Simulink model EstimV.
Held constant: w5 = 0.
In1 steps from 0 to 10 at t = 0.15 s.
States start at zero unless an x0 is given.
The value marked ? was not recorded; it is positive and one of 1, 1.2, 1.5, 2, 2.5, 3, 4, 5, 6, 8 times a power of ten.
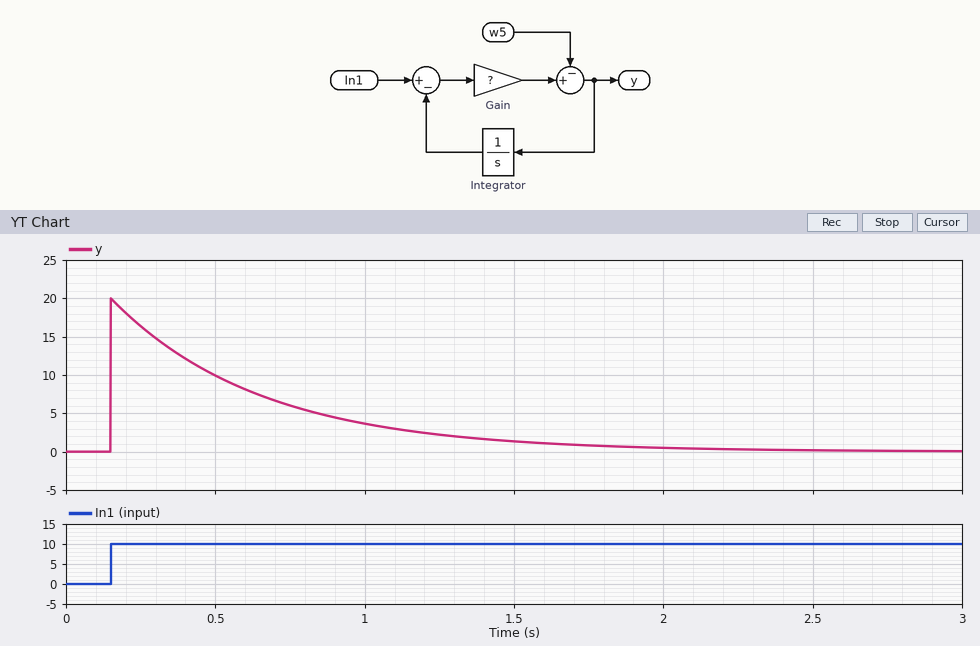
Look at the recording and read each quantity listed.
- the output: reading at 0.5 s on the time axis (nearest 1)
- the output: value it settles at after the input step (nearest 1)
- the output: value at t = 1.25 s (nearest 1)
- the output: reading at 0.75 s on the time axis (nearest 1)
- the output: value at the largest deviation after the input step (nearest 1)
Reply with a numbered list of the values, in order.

1. 10
2. 0
3. 2
4. 6
5. 20
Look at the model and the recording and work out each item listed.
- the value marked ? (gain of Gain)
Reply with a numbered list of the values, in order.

1. 2
